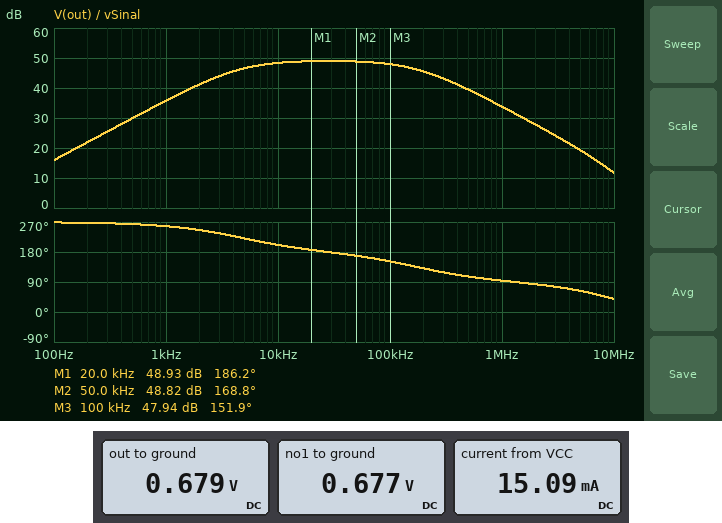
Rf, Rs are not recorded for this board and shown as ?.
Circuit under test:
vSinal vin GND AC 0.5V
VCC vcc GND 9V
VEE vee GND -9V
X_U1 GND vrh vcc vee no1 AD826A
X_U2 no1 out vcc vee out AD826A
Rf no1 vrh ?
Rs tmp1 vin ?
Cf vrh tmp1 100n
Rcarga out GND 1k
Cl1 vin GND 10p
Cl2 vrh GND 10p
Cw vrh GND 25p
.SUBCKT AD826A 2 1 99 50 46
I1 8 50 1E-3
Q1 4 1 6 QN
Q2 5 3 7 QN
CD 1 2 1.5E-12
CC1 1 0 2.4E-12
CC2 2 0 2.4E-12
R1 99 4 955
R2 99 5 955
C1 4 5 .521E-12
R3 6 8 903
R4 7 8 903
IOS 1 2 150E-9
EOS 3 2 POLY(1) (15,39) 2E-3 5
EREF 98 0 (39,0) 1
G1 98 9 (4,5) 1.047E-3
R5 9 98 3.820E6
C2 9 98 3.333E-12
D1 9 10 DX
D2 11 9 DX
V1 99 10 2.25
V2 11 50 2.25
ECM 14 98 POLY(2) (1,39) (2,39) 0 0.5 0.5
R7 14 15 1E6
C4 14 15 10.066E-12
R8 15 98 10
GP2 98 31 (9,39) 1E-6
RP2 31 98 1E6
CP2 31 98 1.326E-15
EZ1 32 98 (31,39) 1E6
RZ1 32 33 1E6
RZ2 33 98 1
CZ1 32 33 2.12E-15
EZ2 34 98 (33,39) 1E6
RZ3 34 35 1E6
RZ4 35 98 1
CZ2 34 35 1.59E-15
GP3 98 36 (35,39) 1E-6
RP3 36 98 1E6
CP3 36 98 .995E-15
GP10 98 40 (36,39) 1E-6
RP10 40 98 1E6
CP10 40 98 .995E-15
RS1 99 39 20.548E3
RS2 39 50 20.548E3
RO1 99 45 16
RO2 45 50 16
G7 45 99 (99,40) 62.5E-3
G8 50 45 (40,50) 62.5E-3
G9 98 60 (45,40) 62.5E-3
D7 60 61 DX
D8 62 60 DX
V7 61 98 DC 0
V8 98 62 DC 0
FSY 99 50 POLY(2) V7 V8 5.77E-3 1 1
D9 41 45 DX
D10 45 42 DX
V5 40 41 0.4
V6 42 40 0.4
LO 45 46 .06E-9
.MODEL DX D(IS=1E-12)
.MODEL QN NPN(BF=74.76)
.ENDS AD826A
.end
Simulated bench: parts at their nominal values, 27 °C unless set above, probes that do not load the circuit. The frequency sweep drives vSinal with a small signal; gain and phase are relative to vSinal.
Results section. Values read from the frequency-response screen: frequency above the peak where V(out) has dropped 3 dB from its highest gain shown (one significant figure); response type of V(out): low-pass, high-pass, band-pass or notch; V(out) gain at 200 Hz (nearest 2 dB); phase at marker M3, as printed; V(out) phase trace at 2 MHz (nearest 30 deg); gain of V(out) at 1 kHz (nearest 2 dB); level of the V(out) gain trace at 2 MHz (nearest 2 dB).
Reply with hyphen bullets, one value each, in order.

- 200 kHz
- band-pass
- 22 dB
- 151.9 deg
- 90 deg
- 36 dB
- 28 dB
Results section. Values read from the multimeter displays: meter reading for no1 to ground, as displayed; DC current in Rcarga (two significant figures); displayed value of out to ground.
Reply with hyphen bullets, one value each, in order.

- 0.677 V
- 680 µA
- 0.679 V
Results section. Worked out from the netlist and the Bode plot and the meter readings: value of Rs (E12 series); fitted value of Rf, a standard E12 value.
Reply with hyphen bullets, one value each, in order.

- 330 Ω
- 100 kΩ
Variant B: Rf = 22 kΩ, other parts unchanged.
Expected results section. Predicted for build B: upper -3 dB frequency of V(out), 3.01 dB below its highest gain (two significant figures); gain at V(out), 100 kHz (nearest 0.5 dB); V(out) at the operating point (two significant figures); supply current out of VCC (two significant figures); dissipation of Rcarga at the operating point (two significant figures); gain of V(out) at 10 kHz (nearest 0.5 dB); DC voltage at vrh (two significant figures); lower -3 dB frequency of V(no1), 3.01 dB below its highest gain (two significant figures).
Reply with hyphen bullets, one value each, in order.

- 790 kHz
- 36.5 dB
- 150 mV
- 15 mA
- 23 µW
- 35.5 dB
- 2.0 mV
- 4.7 kHz
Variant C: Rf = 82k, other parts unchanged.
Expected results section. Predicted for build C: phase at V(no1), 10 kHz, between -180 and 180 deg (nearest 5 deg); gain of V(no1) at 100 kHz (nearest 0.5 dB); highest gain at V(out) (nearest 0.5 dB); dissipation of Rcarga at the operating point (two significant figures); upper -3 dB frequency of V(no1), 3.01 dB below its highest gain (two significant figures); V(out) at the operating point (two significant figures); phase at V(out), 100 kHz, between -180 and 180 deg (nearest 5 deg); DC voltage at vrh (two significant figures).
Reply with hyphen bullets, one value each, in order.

- -160 deg
- 46.5 dB
- 47.5 dB
- 310 µW
- 220 kHz
- 560 mV
- 155 deg
- 1.9 mV
